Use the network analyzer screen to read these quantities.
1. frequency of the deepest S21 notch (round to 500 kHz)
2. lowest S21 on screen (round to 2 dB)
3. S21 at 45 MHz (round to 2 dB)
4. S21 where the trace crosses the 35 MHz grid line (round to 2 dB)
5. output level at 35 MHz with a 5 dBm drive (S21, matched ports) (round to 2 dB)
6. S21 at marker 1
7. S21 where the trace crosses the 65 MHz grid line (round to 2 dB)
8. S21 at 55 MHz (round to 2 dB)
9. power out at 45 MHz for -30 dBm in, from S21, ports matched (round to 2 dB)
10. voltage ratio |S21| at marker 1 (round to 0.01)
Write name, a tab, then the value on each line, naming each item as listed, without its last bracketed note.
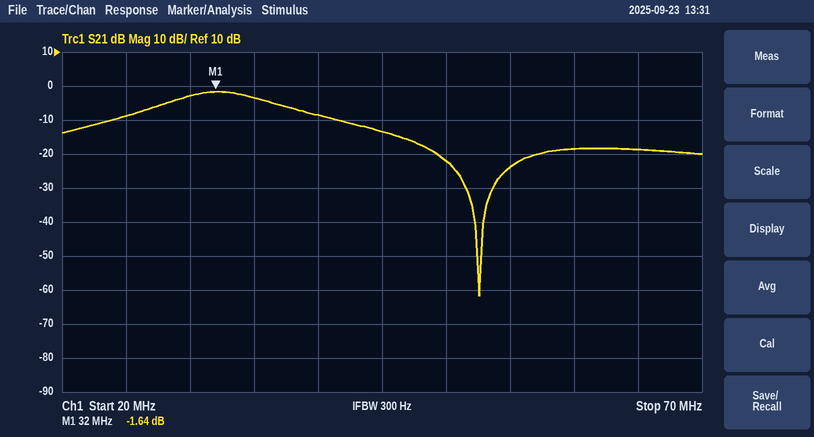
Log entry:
frequency of the deepest S21 notch	52.5 MHz
lowest S21 on screen	-62 dB
S21 at 45 MHz	-14 dB
S21 where the trace crosses the 35 MHz grid line	-4 dB
output level at 35 MHz with a 5 dBm drive (S21, matched ports)	2 dBm
S21 at marker 1	-1.64 dB
S21 where the trace crosses the 65 MHz grid line	-18 dB
S21 at 55 MHz	-24 dB
power out at 45 MHz for -30 dBm in, from S21, ports matched	-44 dBm
voltage ratio |S21| at marker 1	0.83
